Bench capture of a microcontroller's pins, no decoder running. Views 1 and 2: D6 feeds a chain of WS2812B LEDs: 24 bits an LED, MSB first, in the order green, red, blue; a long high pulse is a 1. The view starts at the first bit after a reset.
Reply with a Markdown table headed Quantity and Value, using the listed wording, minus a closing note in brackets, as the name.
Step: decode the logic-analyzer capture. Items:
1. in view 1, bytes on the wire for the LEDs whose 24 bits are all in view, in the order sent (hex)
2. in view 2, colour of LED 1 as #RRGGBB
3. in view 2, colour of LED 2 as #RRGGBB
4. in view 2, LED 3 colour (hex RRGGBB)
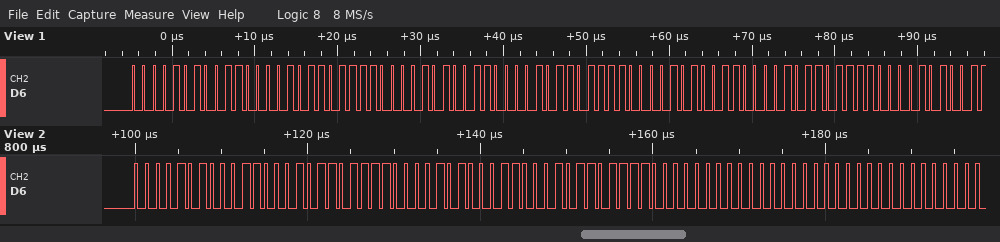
| Quantity | Value |
|---|---|
| in view 1, bytes on the wire for the LEDs whose 24 bits are all in view, in the order sent | 0A 61 6F 0A 61 6F 0A 61 6F |
| in view 2, colour of LED 1 as #RRGGBB | #310A6F |
| in view 2, colour of LED 2 as #RRGGBB | #310A6F |
| in view 2, LED 3 colour | #000000 |
